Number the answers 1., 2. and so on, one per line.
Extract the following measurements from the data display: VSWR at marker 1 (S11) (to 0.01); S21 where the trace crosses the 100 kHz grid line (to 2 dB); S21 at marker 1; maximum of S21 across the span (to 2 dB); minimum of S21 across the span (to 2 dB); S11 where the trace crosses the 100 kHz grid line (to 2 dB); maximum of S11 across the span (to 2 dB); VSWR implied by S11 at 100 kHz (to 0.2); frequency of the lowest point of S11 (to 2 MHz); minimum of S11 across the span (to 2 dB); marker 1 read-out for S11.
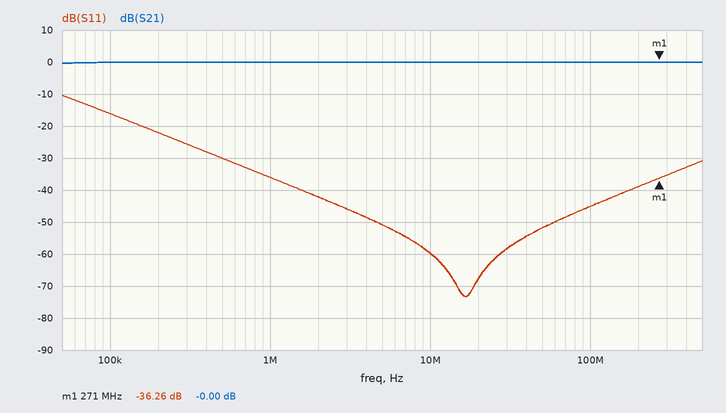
1. 1.03
2. 0 dB
3. -0.00 dB
4. 0 dB
5. 0 dB
6. -16 dB
7. -10 dB
8. 1.4
9. 16 MHz
10. -74 dB
11. -36.26 dB
